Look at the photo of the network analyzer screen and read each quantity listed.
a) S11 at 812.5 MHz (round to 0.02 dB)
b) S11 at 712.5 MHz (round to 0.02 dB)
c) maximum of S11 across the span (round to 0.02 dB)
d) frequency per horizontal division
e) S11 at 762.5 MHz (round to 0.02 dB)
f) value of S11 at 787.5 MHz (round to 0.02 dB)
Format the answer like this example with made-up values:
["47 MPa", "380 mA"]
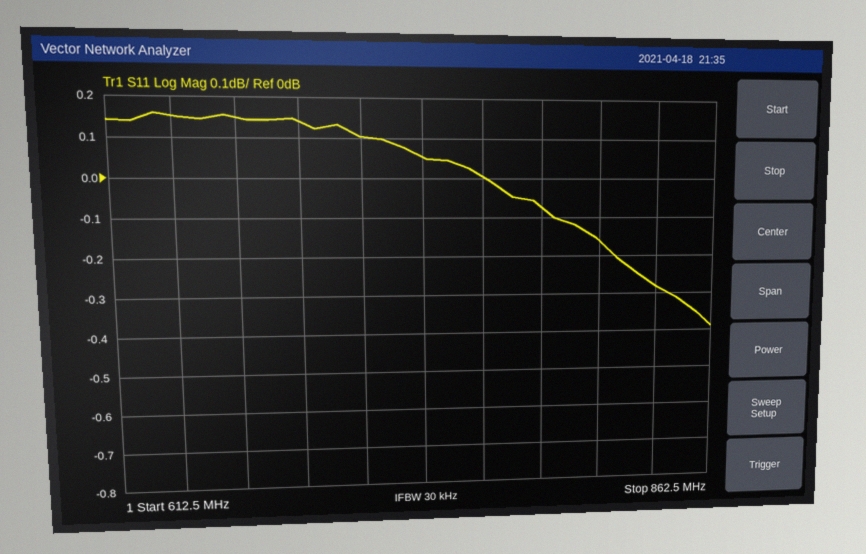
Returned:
["-0.16 dB", "0.10 dB", "0.16 dB", "25 MHz", "0.00 dB", "-0.08 dB"]
